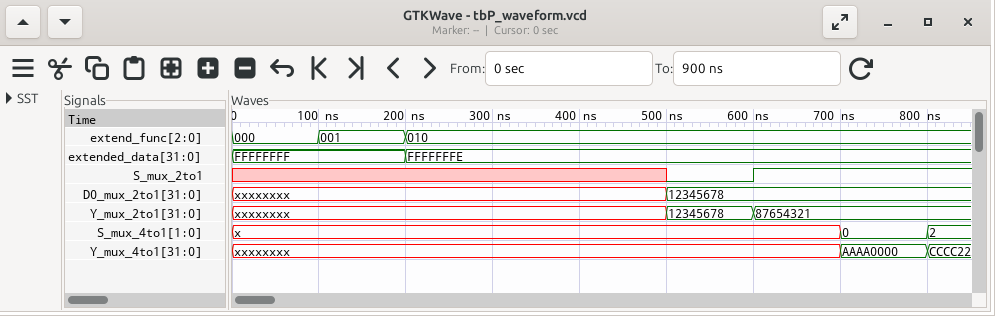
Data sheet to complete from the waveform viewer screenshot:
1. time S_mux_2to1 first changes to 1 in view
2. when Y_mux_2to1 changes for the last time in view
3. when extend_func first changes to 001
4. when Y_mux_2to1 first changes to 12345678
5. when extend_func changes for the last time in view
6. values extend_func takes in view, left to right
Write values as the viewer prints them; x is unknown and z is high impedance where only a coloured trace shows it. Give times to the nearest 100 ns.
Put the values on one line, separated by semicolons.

600 ns; 600 ns; 100 ns; 500 ns; 200 ns; 000, 001, 010
